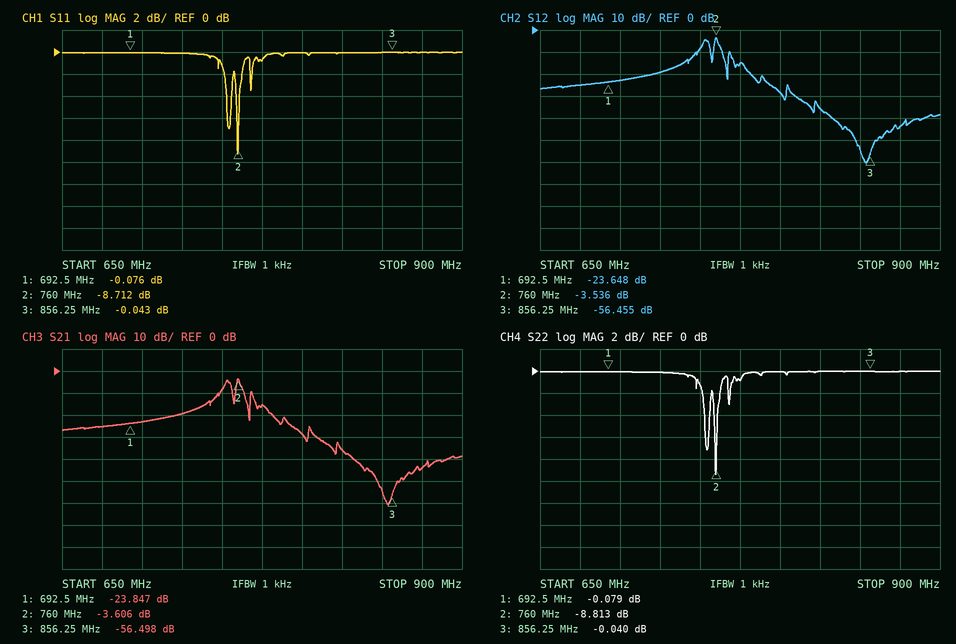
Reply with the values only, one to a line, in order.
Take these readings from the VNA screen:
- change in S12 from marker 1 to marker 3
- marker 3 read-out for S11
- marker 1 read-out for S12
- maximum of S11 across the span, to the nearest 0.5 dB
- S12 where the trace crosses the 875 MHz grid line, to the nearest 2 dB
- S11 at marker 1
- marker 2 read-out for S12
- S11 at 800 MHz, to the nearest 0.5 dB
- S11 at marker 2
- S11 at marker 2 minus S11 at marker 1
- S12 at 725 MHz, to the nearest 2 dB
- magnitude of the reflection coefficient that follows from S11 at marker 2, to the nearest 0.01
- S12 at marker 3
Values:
-32.807 dB
-0.043 dB
-23.648 dB
0.0 dB
-44 dB
-0.076 dB
-3.536 dB
0.0 dB
-8.712 dB
-8.636 dB
-20 dB
0.37
-56.455 dB
